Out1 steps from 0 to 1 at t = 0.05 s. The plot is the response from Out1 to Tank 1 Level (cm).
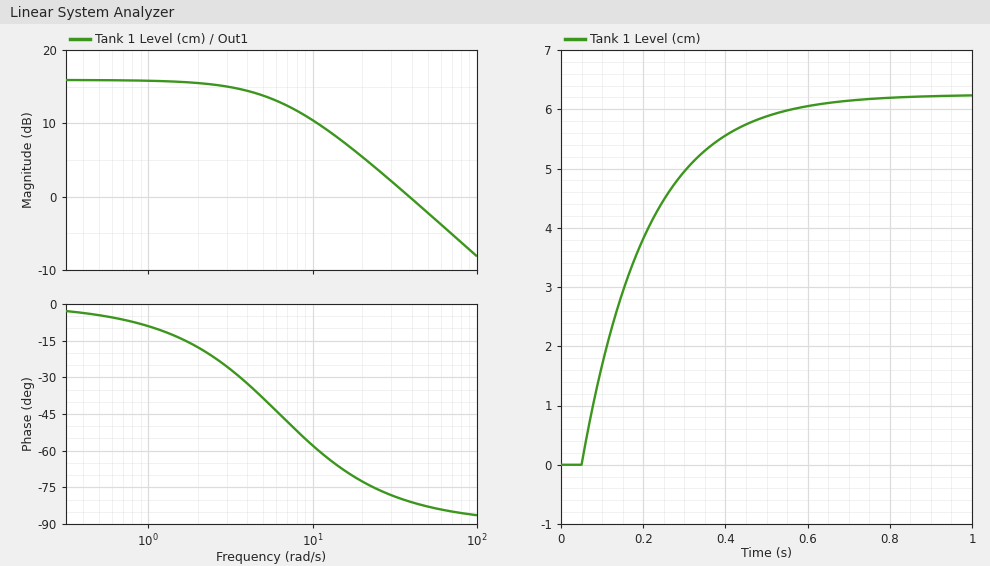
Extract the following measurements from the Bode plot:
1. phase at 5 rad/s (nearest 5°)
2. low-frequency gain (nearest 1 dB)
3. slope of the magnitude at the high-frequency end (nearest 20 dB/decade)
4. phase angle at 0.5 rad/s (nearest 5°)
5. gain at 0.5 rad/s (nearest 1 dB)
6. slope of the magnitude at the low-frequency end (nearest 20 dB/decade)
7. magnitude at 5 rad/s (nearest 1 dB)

-40°
16 dB
-20 dB/decade
-5°
16 dB
0 dB/decade
14 dB
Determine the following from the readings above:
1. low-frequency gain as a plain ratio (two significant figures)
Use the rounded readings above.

6.3
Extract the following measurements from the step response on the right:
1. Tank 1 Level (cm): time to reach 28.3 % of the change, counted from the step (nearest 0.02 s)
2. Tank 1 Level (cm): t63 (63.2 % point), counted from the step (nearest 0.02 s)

0.06 s
0.16 s
